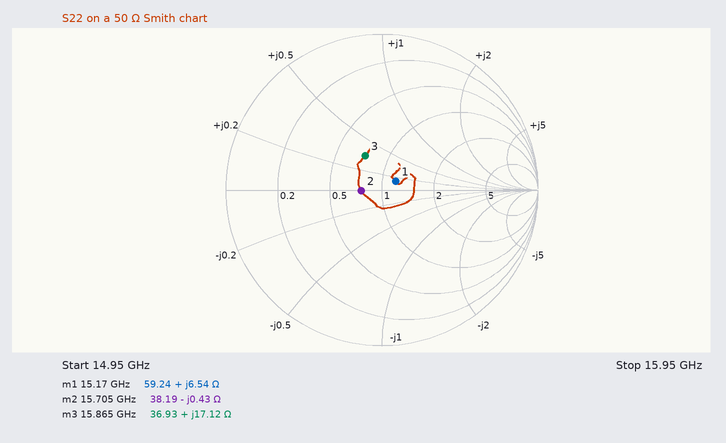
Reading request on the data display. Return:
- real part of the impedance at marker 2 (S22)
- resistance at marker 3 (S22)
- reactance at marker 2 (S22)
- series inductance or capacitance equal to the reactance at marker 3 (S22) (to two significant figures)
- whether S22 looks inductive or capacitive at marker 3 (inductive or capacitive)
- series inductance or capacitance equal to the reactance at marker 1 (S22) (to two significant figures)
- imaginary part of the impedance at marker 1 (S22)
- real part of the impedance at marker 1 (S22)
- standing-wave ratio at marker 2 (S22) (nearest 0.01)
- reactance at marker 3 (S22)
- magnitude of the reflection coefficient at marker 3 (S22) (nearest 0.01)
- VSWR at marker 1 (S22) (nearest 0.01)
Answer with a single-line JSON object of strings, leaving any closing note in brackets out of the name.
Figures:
{"real part of the impedance at marker 2": "38.19 Ω", "resistance at marker 3": "36.93 Ω", "reactance at marker 2": "-0.43 Ω", "series inductance or capacitance equal to the reactance at marker 3 (S22)": "170 pH", "whether S22 looks inductive or capacitive at marker 3": "inductive", "series inductance or capacitance equal to the reactance at marker 1 (S22)": "69 pH", "imaginary part of the impedance at marker 1": "+6.54 Ω", "real part of the impedance at marker 1": "59.24 Ω", "standing-wave ratio at marker 2 (S22)": "1.31", "reactance at marker 3": "+17.12 Ω", "magnitude of the reflection coefficient at marker 3 (S22)": "0.24", "VSWR at marker 1 (S22)": "1.23"}
